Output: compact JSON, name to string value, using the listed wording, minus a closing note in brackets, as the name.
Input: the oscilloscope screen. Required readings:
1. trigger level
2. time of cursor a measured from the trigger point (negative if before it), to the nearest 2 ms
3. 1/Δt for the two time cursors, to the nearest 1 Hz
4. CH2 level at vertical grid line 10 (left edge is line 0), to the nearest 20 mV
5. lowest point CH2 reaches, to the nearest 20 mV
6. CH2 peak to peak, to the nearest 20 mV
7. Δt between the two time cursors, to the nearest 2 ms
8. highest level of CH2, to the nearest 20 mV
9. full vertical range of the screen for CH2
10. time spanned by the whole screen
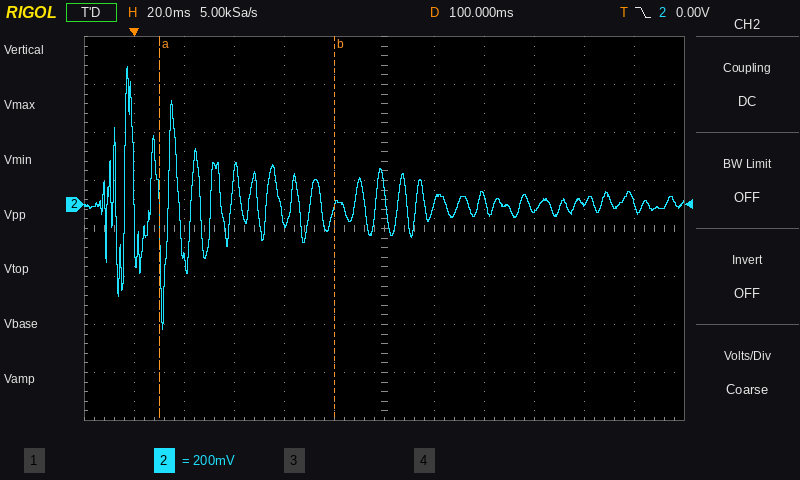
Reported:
{"trigger level": "0.00 V", "time of cursor a measured from the trigger point (negative if before it), to the nearest 2 ms": "+10 ms", "1/Δt for the two time cursors, to the nearest 1 Hz": "14 Hz", "CH2 level at vertical grid line 10 (left edge is line 0), to the nearest 20 mV": "0 mV", "lowest point CH2 reaches, to the nearest 20 mV": "-520 mV", "CH2 peak to peak, to the nearest 20 mV": "1.10 V", "Δt between the two time cursors, to the nearest 2 ms": "70 ms", "highest level of CH2, to the nearest 20 mV": "580 mV", "full vertical range of the screen for CH2": "1.6 V", "time spanned by the whole screen": "240 ms"}
